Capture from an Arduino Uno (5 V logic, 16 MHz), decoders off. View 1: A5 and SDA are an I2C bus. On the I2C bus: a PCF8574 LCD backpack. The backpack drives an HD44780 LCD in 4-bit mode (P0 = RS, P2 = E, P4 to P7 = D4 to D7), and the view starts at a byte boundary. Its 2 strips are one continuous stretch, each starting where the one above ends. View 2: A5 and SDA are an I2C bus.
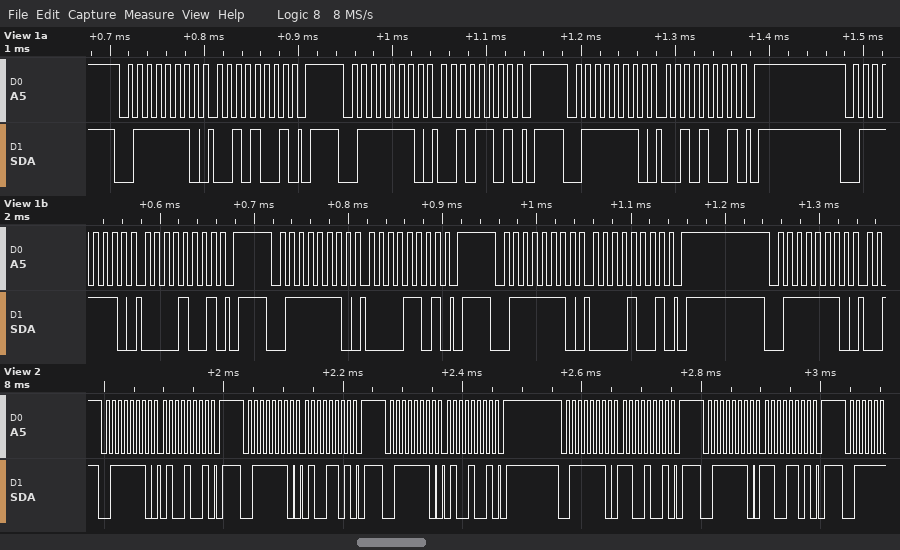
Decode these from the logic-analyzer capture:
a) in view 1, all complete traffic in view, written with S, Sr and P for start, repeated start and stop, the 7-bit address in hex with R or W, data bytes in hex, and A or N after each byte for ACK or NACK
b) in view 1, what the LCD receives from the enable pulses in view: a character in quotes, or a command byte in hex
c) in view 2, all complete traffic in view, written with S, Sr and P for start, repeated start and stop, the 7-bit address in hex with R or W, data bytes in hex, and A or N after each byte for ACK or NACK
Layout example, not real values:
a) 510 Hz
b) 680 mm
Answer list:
a) S 3FW A 29 A P S 3FW A 2D A P S 3FW A 29 A P S 3FW A 09 A P S 3FW A 0D A P S 3FW A 09 A P S 3FW A
b) ' '
c) S 3FW A 49 A P S 3FW A 4D A P S 3FW A 49 A P S 3FW A C9 A P S 3FW A CD A P
